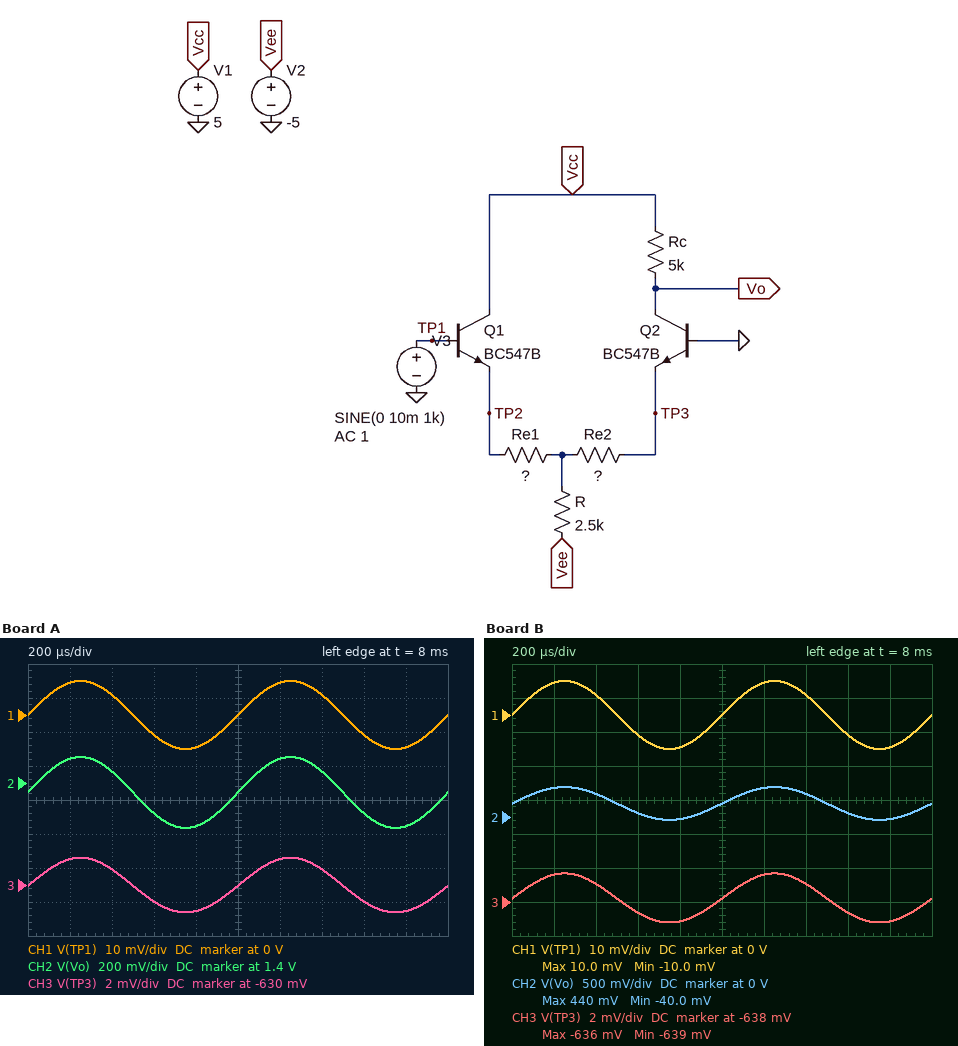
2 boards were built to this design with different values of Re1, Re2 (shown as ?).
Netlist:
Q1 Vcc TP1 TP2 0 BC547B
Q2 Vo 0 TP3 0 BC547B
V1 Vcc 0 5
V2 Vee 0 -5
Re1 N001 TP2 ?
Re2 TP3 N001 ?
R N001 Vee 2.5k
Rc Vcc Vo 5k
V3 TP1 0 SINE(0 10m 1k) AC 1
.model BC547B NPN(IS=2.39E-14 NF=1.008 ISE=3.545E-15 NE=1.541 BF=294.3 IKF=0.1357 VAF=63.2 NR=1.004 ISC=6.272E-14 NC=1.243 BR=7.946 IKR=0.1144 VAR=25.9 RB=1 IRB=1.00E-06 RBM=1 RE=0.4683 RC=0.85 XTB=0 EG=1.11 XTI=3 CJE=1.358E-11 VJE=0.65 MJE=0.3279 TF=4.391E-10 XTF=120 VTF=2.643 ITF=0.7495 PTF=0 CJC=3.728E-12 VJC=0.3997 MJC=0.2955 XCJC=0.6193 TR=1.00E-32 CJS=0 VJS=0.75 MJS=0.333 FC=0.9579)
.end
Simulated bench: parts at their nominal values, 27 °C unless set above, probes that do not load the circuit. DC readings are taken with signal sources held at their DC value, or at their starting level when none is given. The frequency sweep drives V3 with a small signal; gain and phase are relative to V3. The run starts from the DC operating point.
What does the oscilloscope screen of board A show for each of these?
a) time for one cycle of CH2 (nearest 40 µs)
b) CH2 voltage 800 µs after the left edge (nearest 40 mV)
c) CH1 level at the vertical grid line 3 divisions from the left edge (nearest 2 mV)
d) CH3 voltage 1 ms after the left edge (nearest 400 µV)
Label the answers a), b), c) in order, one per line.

a) 1.00 ms
b) 1.16 V
c) -6 mV
d) -630.0 mV
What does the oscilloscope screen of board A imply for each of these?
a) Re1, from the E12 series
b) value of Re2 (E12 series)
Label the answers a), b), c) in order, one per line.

a) 68 Ω
b) 100 Ω
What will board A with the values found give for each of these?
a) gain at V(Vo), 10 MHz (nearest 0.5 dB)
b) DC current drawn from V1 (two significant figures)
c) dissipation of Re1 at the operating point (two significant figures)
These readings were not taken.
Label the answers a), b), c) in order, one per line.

a) 24.5 dB
b) 1.7 mA
c) 66 µW
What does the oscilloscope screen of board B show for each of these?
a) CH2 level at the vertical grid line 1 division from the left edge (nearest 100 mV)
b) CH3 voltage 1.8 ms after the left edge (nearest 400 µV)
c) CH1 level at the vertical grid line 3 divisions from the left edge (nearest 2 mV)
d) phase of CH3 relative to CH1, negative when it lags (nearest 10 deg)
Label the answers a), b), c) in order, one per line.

a) 400 mV
b) -639.2 mV
c) -6 mV
d) 0 deg
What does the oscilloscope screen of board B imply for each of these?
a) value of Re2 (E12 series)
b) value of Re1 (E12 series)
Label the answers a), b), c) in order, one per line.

a) 56 Ω
b) 82 Ω
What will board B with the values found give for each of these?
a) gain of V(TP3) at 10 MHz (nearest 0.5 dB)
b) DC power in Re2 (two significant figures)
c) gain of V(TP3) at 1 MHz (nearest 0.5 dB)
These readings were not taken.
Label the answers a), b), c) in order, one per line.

a) -17.0 dB
b) 52 µW
c) -17.0 dB
